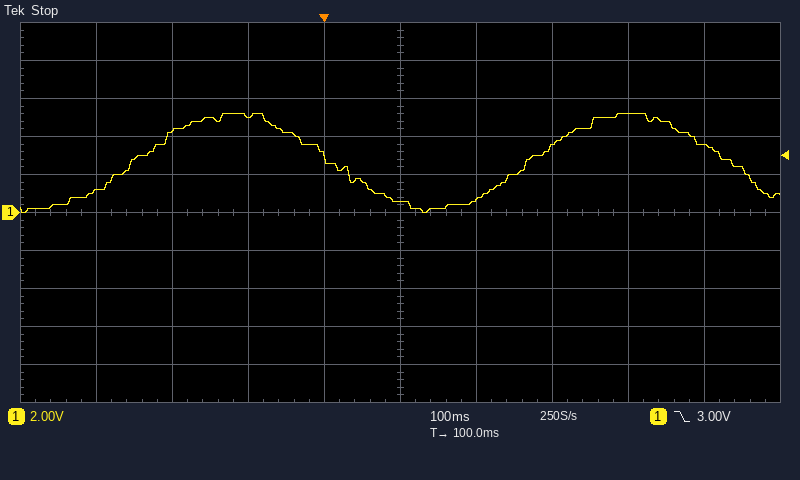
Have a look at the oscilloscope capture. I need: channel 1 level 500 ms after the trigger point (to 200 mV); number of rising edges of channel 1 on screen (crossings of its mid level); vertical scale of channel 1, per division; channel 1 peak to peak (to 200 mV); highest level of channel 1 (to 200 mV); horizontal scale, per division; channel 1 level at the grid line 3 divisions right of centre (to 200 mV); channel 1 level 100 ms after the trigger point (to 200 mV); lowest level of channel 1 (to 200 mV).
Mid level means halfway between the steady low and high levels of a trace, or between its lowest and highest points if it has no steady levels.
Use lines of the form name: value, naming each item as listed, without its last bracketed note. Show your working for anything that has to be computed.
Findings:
channel 1 level 500 ms after the trigger point: 3.6 V
number of rising edges of channel 1 on screen: 2
vertical scale of channel 1, per division: 2 V
channel 1 peak to peak: 5.2 V − (0.0 V) = 5.2 V
highest level of channel 1: 5.2 V
horizontal scale, per division: 100 ms
channel 1 level at the grid line 3 divisions right of centre: 5.2 V
channel 1 level 100 ms after the trigger point: 600 mV
lowest level of channel 1: 0.0 V
